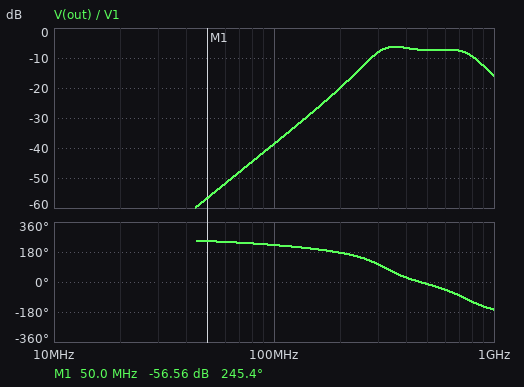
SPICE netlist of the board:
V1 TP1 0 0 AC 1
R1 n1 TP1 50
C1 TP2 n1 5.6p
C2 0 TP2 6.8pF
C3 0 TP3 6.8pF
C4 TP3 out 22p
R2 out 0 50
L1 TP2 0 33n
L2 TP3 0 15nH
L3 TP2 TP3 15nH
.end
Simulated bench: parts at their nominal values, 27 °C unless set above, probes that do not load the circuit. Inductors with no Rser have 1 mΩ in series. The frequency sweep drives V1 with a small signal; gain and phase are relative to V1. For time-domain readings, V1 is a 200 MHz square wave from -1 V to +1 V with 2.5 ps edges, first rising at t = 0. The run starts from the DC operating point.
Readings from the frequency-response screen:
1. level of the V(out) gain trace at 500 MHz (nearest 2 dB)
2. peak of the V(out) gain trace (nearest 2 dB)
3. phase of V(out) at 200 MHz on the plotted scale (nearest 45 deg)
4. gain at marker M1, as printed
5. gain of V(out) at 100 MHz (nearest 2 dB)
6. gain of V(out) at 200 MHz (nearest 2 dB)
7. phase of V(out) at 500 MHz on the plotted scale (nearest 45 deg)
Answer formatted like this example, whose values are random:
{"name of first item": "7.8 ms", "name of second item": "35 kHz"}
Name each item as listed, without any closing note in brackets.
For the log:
{"level of the V(out) gain trace at 500 MHz": "-8 dB", "peak of the V(out) gain trace": "-6 dB", "phase of V(out) at 200 MHz on the plotted scale": "180 deg", "gain at marker M1, as printed": "-56.56 dB", "gain of V(out) at 100 MHz": "-38 dB", "gain of V(out) at 200 MHz": "-20 dB", "phase of V(out) at 500 MHz on the plotted scale": "0 deg"}
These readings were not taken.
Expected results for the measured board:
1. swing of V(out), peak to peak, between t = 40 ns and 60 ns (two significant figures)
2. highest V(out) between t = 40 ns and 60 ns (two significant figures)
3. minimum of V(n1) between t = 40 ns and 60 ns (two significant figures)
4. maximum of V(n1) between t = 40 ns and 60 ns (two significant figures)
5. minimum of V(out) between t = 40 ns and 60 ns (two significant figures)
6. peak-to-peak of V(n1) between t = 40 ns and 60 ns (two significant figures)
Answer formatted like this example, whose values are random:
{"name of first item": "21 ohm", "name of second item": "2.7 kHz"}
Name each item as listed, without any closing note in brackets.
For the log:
{"swing of V(out), peak to peak, between t = 40 ns and 60 ns": "630 mV", "highest V(out) between t = 40 ns and 60 ns": "320 mV", "minimum of V(n1) between t = 40 ns and 60 ns": "-1.1 V", "maximum of V(n1) between t = 40 ns and 60 ns": "1.1 V", "minimum of V(out) between t = 40 ns and 60 ns": "-320 mV", "peak-to-peak of V(n1) between t = 40 ns and 60 ns": "2.2 V"}
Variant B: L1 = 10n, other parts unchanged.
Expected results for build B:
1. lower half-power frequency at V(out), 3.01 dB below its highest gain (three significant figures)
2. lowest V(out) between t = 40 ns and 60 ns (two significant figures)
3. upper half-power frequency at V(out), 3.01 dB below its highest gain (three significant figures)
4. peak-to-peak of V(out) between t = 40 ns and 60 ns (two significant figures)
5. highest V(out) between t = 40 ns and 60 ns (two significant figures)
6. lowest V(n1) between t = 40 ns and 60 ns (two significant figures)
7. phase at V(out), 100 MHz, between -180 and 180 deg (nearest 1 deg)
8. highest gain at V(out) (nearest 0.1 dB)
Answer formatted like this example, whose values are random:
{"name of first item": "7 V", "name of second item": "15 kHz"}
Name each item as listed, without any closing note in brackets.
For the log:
{"lower half-power frequency at V(out), 3.01 dB below its highest gain": "429 MHz", "lowest V(out) between t = 40 ns and 60 ns": "-290 mV", "upper half-power frequency at V(out), 3.01 dB below its highest gain": "875 MHz", "peak-to-peak of V(out) between t = 40 ns and 60 ns": "580 mV", "highest V(out) between t = 40 ns and 60 ns": "290 mV", "lowest V(n1) between t = 40 ns and 60 ns": "-1.1 V", "phase at V(out), 100 MHz, between -180 and 180 deg": "-137 deg", "highest gain at V(out)": "-6.0 dB"}
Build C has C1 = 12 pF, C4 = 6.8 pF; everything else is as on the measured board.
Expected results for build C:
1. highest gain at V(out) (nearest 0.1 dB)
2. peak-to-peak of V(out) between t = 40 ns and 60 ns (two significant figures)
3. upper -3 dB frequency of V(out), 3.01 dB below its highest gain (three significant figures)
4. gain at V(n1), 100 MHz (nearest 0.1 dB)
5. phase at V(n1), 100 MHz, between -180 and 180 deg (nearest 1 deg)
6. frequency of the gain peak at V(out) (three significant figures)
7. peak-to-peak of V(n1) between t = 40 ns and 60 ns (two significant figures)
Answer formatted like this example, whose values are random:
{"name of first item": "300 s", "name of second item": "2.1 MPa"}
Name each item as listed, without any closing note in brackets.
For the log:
{"highest gain at V(out)": "-6.1 dB", "peak-to-peak of V(out) between t = 40 ns and 60 ns": "660 mV", "upper -3 dB frequency of V(out), 3.01 dB below its highest gain": "802 MHz", "gain at V(n1), 100 MHz": "-0.7 dB", "phase at V(n1), 100 MHz, between -180 and 180 deg": "-22 deg", "frequency of the gain peak at V(out)": "650 MHz", "peak-to-peak of V(n1) between t = 40 ns and 60 ns": "2.3 V"}
